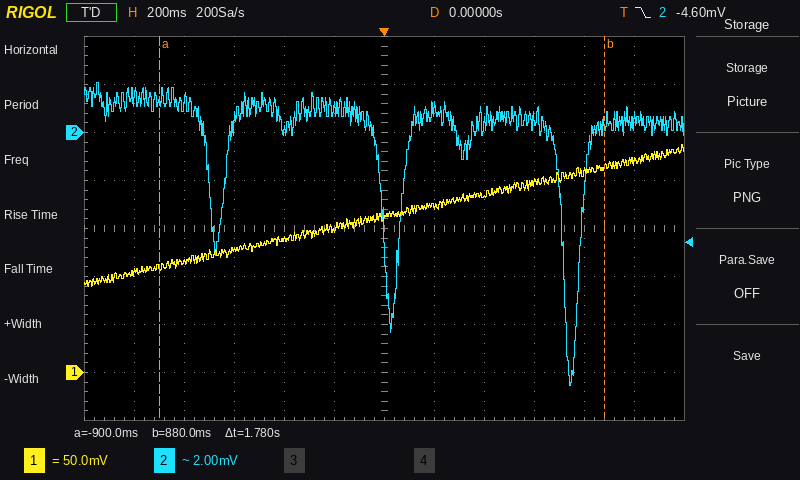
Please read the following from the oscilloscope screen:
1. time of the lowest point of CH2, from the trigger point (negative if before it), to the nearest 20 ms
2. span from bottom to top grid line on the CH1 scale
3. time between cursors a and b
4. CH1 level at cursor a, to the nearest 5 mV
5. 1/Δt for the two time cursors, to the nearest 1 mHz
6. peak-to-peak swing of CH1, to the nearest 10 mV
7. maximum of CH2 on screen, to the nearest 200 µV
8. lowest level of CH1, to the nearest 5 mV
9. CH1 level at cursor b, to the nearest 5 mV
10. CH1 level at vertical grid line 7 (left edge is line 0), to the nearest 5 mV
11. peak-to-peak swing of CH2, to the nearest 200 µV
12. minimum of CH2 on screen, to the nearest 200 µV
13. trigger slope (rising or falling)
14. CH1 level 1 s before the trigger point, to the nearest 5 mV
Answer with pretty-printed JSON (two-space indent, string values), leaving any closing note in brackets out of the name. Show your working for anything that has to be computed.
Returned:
{
  "time of the lowest point of CH2, from the trigger point (negative if before it), to the nearest 20 ms": "+740 ms",
  "span from bottom to top grid line on the CH1 scale": "400 mV",
  "time between cursors a and b": "1.78 s",
  "CH1 level at cursor a, to the nearest 5 mV": "110 mV",
  "1/Δt for the two time cursors, to the nearest 1 mHz": "1 / 1.78 s ≈ 562 mHz",
  "peak-to-peak swing of CH1, to the nearest 10 mV": "150 mV",
  "maximum of CH2 on screen, to the nearest 200 µV": "2.0 mV",
  "lowest level of CH1, to the nearest 5 mV": "90 mV",
  "CH1 level at cursor b, to the nearest 5 mV": "215 mV",
  "CH1 level at vertical grid line 7 (left edge is line 0), to the nearest 5 mV": "175 mV",
  "peak-to-peak swing of CH2, to the nearest 200 µV": "2.0 mV − (-10.6 mV) = 12.6 mV",
  "minimum of CH2 on screen, to the nearest 200 µV": "-10.6 mV",
  "trigger slope": "falling",
  "CH1 level 1 s before the trigger point, to the nearest 5 mV": "105 mV"
}
